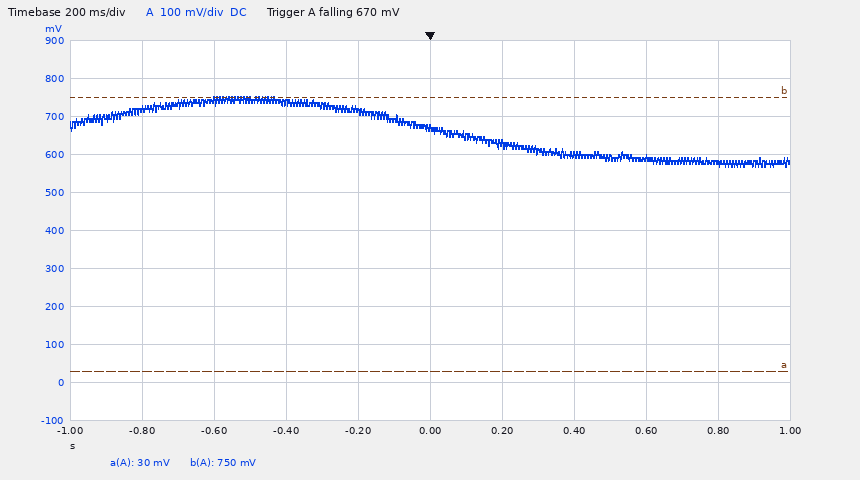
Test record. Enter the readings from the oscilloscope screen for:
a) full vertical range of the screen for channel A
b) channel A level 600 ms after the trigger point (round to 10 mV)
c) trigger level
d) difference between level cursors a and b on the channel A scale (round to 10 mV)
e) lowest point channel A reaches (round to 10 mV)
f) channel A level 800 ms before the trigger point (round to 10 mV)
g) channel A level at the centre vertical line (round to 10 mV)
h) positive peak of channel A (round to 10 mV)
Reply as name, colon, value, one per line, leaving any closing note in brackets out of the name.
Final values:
full vertical range of the screen for channel A: 1 V
channel A level 600 ms after the trigger point: 590 mV
trigger level: 670 mV
difference between level cursors a and b on the channel A scale: 720 mV
lowest point channel A reaches: 570 mV
channel A level 800 ms before the trigger point: 720 mV
channel A level at the centre vertical line: 670 mV
positive peak of channel A: 750 mV
